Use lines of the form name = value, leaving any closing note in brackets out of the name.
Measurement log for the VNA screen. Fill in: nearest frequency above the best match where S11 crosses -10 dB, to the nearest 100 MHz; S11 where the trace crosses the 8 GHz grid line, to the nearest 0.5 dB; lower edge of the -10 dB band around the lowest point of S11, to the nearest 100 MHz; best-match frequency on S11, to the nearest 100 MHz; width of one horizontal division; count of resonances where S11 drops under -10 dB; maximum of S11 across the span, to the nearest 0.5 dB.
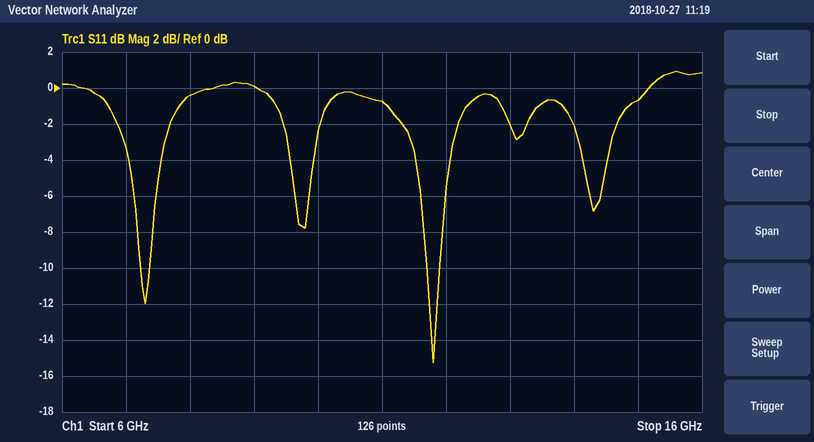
nearest frequency above the best match where S11 crosses -10 dB, to the nearest 100 MHz = 11.9 GHz
S11 where the trace crosses the 8 GHz grid line, to the nearest 0.5 dB = -0.5 dB
lower edge of the -10 dB band around the lowest point of S11, to the nearest 100 MHz = 11.7 GHz
best-match frequency on S11, to the nearest 100 MHz = 11.8 GHz
width of one horizontal division = 1 GHz
count of resonances where S11 drops under -10 dB = 2
maximum of S11 across the span, to the nearest 0.5 dB = 1.0 dB
